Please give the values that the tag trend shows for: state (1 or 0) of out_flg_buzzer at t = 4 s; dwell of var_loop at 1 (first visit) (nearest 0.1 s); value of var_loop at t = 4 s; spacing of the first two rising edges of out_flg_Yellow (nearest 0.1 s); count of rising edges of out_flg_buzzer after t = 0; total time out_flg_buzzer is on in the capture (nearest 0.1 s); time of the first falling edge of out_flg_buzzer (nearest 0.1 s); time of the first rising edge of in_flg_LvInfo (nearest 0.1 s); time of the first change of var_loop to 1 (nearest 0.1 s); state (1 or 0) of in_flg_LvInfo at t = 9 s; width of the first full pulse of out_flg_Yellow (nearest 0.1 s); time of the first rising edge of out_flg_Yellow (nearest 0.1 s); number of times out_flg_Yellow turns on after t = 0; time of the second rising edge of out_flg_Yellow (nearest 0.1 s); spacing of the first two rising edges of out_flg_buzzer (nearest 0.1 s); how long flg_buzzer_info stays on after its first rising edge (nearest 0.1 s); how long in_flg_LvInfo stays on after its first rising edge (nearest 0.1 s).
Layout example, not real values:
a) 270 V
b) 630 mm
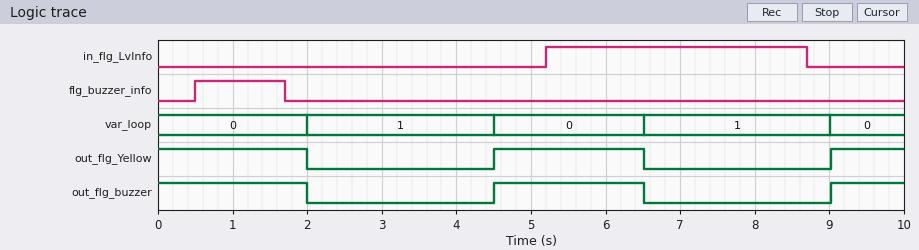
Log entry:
a) 0
b) 2.5 s
c) 1
d) 4.5 s
e) 2
f) 5.0 s
g) 2.0 s
h) 5.2 s
i) 2.0 s
j) 0
k) 2.0 s
l) 4.5 s
m) 2
n) 9.0 s
o) 4.5 s
p) 1.2 s
q) 3.5 s
